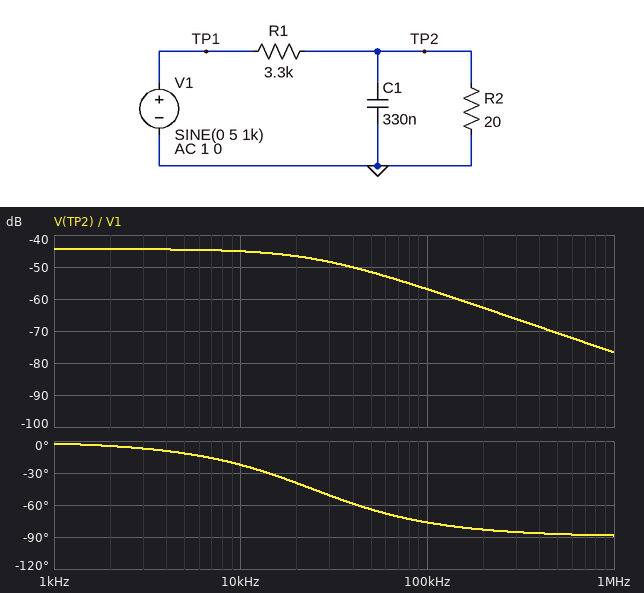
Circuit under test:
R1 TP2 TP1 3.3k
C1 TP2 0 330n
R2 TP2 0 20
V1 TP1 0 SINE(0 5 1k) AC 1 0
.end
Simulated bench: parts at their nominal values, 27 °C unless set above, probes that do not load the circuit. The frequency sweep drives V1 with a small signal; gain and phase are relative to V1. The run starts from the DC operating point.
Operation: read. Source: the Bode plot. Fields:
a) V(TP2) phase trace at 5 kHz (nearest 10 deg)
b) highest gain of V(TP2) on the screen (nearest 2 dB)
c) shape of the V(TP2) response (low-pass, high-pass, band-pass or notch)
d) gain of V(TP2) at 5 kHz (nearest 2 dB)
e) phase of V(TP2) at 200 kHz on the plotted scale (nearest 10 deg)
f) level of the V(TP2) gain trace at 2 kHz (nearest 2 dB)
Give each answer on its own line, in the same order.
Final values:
-10 deg
-44 dB
low-pass
-44 dB
-80 deg
-44 dB
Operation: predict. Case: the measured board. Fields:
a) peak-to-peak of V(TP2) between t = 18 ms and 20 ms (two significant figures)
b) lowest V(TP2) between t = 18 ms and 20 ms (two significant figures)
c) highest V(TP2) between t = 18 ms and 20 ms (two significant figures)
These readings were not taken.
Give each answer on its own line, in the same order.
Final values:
60 mV
-30 mV
30 mV
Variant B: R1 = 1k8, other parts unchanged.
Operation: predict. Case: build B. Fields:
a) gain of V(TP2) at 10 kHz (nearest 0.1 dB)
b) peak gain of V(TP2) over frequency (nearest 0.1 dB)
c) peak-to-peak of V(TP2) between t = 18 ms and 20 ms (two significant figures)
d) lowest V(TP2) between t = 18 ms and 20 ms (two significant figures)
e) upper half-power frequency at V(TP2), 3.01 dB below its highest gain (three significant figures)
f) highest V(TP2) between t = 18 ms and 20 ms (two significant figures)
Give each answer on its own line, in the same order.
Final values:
-39.9 dB
-39.2 dB
110 mV
-55 mV
24.4 kHz
55 mV
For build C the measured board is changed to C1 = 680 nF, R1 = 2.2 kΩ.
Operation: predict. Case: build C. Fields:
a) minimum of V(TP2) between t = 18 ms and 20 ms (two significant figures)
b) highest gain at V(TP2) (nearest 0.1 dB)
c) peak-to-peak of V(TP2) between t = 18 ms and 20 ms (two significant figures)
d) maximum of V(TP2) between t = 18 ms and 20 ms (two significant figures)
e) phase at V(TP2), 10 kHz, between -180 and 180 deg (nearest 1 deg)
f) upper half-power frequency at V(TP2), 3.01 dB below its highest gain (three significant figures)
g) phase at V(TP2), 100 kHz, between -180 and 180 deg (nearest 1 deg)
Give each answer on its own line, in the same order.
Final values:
-45 mV
-40.9 dB
90 mV
45 mV
-40 deg
11.8 kHz
-83 deg
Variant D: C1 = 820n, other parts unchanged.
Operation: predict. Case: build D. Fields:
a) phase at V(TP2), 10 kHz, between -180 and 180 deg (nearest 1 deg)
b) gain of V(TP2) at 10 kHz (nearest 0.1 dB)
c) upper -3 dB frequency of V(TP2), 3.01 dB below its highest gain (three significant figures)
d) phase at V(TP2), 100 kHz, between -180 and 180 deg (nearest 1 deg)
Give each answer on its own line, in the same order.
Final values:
-46 deg
-47.5 dB
9.76 kHz
-84 deg
